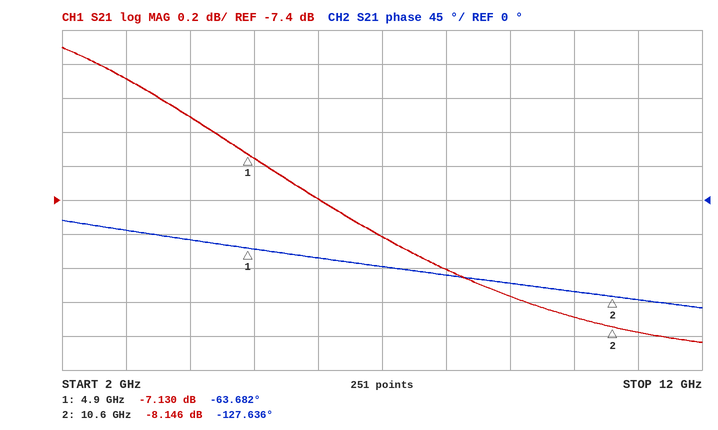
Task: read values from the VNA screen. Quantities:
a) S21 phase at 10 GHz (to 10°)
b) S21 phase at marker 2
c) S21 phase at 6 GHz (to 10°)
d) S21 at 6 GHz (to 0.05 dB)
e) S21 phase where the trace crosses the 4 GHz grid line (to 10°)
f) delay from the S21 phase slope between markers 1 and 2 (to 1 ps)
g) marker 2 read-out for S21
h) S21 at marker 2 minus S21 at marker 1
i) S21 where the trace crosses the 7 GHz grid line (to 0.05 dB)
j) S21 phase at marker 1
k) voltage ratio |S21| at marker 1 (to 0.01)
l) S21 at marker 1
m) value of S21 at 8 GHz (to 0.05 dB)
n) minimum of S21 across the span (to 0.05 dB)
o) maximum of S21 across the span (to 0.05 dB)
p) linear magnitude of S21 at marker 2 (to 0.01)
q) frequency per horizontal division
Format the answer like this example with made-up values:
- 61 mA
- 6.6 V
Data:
- -120°
- -127.636°
- -80°
- -7.40 dB
- -50°
- 31 ps
- -8.146 dB
- -1.016 dB
- -7.60 dB
- -63.682°
- 0.44
- -7.130 dB
- -7.80 dB
- -8.25 dB
- -6.50 dB
- 0.39
- 1 GHz
